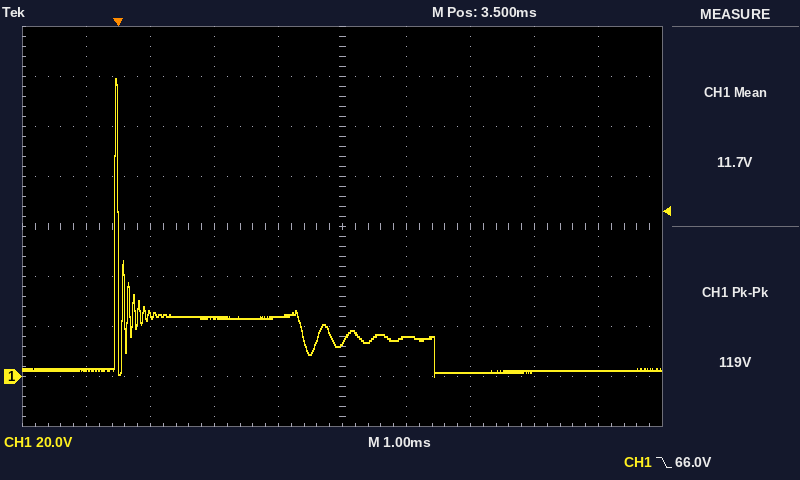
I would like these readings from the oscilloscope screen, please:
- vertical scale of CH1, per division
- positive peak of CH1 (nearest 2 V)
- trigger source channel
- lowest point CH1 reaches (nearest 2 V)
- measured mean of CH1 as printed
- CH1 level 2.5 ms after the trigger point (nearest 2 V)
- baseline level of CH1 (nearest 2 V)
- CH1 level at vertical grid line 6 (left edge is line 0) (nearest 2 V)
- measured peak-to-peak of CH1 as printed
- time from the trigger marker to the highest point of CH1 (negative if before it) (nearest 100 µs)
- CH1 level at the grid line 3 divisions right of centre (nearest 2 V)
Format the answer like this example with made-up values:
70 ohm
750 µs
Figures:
20 V
120 V
CH1
0 V
11.7 V
24 V
2 V
16 V
119 V
0.0 ms
2 V
